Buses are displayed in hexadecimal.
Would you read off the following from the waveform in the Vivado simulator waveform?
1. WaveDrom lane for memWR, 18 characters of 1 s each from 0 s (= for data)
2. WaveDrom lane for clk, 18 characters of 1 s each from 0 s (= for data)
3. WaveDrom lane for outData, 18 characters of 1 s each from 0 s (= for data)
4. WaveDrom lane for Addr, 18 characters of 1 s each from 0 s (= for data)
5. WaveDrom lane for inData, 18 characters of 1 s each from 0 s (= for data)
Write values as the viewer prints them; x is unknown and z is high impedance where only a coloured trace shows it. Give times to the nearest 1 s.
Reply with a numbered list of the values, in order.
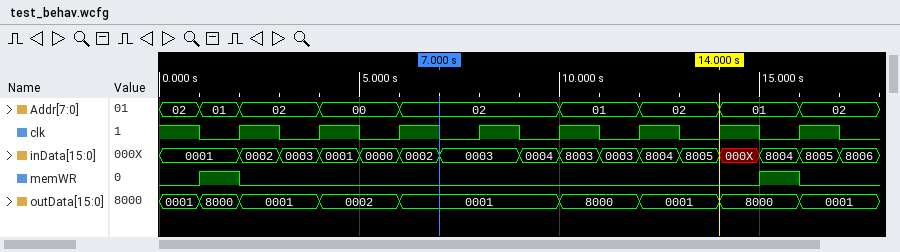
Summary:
1. {name: 'memWR', wave: '010............10.'}
2. {name: 'clk', wave: '101010101010101010'}
3. {name: 'outData', wave: '===.=.=...=.=.=.=.', data: '0001 8000 0001 0002 0001 8000 0001 8000 0001'}
4. {name: 'Addr', wave: '===.=.=...=.=.=.=.', data: '02 01 02 00 02 01 02 01 02'}
5. {name: 'inData', wave: '=.======.=========', data: '0001 0002 0003 0001 0000 0002 0003 0004 8003 0003 8004 8005 000X 8004 8005 8006'}
